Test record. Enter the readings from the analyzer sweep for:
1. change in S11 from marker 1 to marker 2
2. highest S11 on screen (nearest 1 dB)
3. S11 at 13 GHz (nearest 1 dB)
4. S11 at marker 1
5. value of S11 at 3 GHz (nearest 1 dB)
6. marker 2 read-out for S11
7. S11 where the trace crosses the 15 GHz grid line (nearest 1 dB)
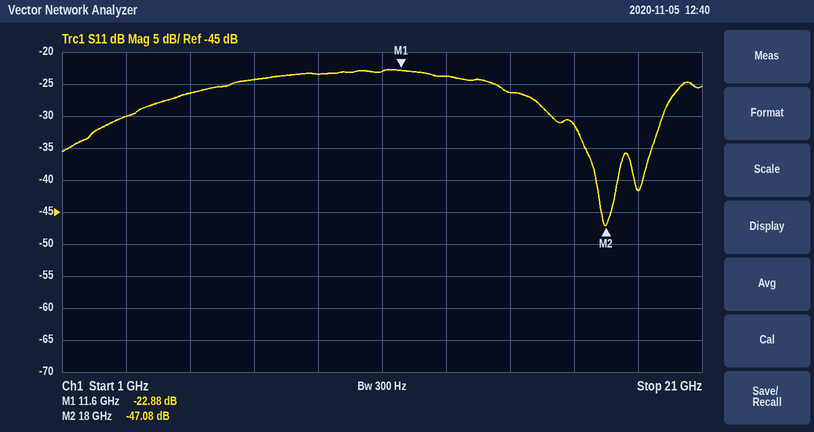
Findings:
-24.20 dB
-23 dB
-24 dB
-22.88 dB
-30 dB
-47.08 dB
-26 dB
